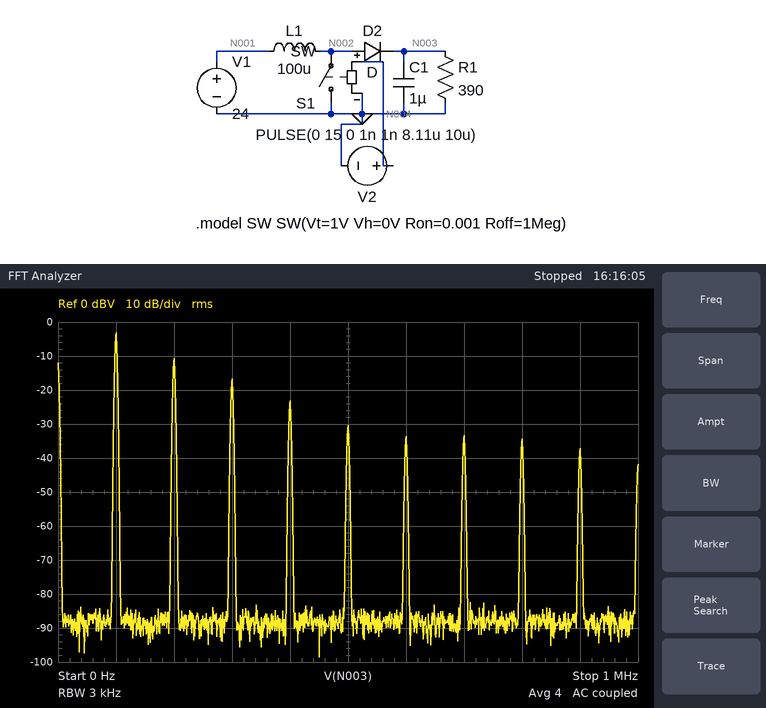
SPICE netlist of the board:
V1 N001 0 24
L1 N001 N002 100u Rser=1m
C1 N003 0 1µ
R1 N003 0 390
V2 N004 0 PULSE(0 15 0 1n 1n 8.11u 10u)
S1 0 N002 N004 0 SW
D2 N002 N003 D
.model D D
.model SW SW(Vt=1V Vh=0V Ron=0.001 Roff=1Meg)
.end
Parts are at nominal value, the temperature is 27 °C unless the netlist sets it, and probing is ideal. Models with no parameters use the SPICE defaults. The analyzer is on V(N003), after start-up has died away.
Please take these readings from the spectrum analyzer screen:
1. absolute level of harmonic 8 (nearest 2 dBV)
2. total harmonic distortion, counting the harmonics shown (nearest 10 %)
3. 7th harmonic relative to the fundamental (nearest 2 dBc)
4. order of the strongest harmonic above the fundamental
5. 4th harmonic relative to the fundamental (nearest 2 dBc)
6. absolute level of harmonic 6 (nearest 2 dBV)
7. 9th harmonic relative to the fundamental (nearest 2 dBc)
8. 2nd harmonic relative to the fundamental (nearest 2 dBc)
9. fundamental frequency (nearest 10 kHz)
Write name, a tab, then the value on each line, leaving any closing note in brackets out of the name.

absolute level of harmonic 8	-34 dBV
total harmonic distortion, counting the harmonics shown	50 %
7th harmonic relative to the fundamental	-30 dBc
order of the strongest harmonic above the fundamental	2
4th harmonic relative to the fundamental	-20 dBc
absolute level of harmonic 6	-34 dBV
9th harmonic relative to the fundamental	-34 dBc
2nd harmonic relative to the fundamental	-8 dBc
fundamental frequency	100 kHz
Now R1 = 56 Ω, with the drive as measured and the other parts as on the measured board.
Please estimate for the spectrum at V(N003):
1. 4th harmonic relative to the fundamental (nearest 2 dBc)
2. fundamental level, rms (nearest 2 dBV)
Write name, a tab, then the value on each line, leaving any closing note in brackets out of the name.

4th harmonic relative to the fundamental	-22 dBc
fundamental level, rms	14 dBV
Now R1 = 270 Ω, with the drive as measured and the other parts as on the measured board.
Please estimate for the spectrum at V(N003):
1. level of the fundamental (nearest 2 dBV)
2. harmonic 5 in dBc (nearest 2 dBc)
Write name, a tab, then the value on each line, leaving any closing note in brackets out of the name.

level of the fundamental	0 dBV
harmonic 5 in dBc	-30 dBc
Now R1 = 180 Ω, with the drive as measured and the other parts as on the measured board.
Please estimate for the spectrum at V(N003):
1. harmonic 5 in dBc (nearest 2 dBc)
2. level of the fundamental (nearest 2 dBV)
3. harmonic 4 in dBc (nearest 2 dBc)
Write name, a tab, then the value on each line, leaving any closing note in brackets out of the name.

harmonic 5 in dBc	-32 dBc
level of the fundamental	4 dBV
harmonic 4 in dBc	-22 dBc
